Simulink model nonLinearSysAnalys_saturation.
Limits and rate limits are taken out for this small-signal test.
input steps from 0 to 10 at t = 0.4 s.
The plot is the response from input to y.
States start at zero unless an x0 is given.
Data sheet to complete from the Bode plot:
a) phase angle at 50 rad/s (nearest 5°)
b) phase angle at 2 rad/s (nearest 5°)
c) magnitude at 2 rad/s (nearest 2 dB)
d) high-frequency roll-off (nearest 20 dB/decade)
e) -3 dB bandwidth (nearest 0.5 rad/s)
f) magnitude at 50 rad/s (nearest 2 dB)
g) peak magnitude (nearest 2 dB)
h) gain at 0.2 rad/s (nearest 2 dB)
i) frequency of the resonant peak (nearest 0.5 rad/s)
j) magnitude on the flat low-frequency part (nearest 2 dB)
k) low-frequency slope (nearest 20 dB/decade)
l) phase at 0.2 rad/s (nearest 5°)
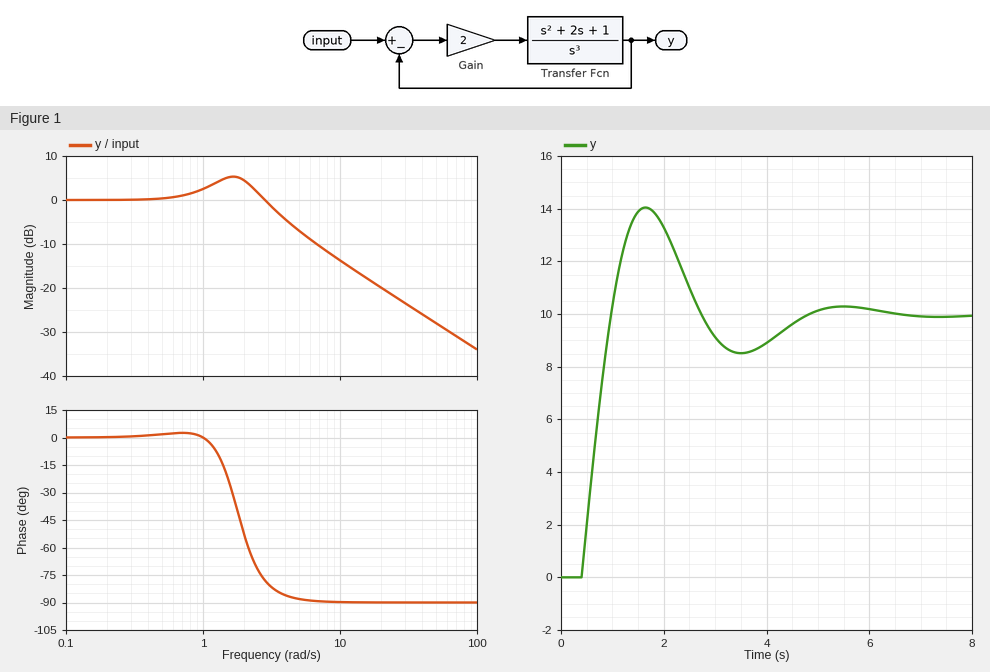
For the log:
-90°
-55°
4 dB
-20 dB/decade
3.5 rad/s
-28 dB
6 dB
0 dB
1.5 rad/s
0 dB
0 dB/decade
0°
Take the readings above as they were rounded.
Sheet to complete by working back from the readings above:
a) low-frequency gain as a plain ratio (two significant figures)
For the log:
1.0
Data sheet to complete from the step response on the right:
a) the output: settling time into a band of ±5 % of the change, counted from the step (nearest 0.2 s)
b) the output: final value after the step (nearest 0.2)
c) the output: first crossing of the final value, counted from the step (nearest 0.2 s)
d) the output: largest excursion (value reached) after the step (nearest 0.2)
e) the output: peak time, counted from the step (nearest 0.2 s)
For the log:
4.0 s
10.0
0.6 s
14.0
1.2 s
